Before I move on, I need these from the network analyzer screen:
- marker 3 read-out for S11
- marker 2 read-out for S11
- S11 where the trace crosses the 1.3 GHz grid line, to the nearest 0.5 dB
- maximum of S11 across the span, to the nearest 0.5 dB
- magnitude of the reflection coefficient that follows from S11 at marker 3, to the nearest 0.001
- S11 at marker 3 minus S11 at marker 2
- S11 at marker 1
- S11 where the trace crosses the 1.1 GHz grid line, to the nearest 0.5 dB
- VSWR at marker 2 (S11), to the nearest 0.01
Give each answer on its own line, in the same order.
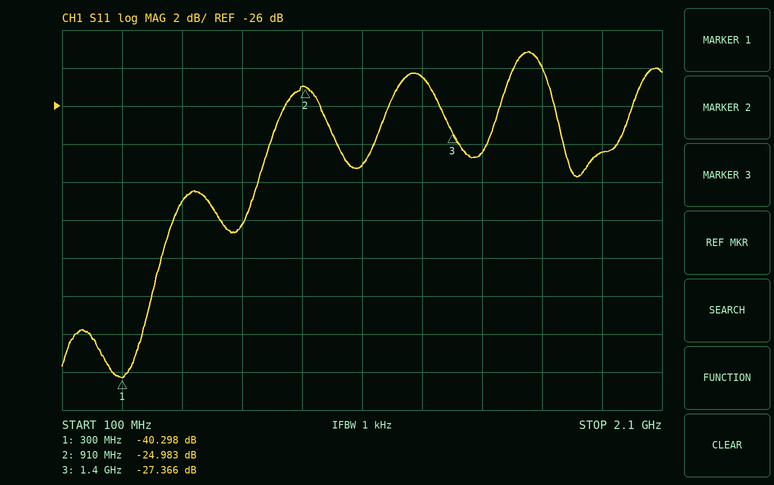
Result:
-27.366 dB
-24.983 dB
-24.5 dB
-23.0 dB
0.043
-2.383 dB
-40.298 dB
-29.0 dB
1.12
